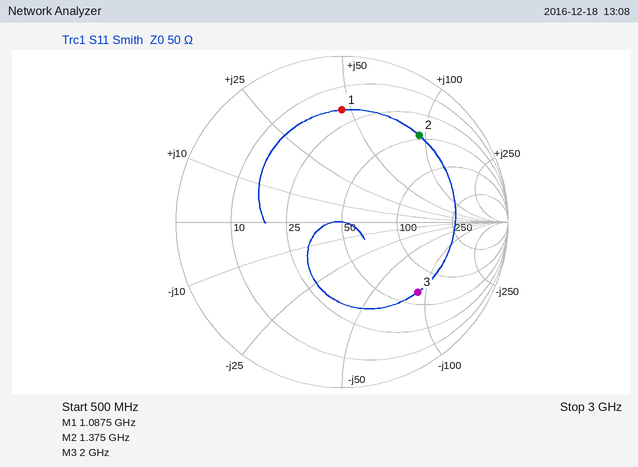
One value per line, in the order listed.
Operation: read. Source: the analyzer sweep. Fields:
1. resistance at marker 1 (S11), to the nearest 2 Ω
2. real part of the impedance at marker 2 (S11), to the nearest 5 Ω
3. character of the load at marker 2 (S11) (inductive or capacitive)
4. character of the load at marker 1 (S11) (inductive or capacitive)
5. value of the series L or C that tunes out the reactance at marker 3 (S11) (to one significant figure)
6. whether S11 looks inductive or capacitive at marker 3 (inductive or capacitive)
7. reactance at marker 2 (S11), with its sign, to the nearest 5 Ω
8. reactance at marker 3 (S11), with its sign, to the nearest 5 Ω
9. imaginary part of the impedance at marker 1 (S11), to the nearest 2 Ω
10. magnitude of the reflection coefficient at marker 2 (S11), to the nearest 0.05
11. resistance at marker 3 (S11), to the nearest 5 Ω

18 Ω
45 Ω
inductive
inductive
7 nH
capacitive
+95 Ω
-90 Ω
+46 Ω
0.70
65 Ω
